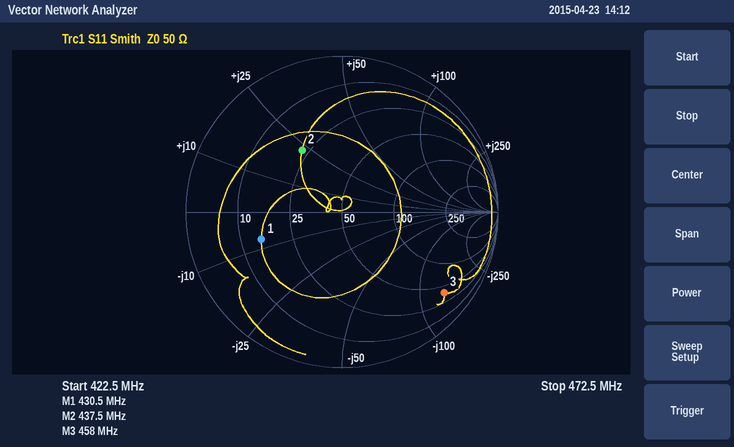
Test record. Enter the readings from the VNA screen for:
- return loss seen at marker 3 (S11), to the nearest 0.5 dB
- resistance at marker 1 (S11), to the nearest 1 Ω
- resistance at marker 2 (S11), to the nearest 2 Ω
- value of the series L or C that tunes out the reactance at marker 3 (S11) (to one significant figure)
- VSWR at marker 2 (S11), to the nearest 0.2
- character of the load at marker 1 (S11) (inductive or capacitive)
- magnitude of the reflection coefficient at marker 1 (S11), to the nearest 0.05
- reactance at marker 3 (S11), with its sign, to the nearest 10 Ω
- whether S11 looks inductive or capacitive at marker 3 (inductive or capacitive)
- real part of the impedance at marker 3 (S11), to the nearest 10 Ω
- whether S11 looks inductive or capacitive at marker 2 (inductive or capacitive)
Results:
1.5 dB
15 Ω
22 Ω
50 nH
2.8
capacitive
0.55
-130 Ω
capacitive
40 Ω
inductive
